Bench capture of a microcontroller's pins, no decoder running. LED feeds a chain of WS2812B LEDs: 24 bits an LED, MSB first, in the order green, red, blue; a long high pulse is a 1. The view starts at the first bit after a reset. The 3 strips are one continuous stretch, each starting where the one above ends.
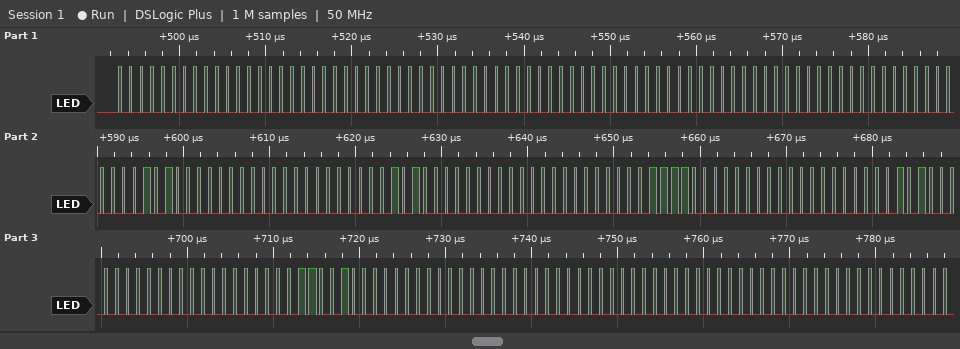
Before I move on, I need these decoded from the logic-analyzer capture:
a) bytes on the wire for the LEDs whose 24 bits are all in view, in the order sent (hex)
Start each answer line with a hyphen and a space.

- 00 00 00 00 00 00 00 00 00 00 28 00 00 50 00 00 78 00 00 A0 00 00 C8 00 00 00 00
